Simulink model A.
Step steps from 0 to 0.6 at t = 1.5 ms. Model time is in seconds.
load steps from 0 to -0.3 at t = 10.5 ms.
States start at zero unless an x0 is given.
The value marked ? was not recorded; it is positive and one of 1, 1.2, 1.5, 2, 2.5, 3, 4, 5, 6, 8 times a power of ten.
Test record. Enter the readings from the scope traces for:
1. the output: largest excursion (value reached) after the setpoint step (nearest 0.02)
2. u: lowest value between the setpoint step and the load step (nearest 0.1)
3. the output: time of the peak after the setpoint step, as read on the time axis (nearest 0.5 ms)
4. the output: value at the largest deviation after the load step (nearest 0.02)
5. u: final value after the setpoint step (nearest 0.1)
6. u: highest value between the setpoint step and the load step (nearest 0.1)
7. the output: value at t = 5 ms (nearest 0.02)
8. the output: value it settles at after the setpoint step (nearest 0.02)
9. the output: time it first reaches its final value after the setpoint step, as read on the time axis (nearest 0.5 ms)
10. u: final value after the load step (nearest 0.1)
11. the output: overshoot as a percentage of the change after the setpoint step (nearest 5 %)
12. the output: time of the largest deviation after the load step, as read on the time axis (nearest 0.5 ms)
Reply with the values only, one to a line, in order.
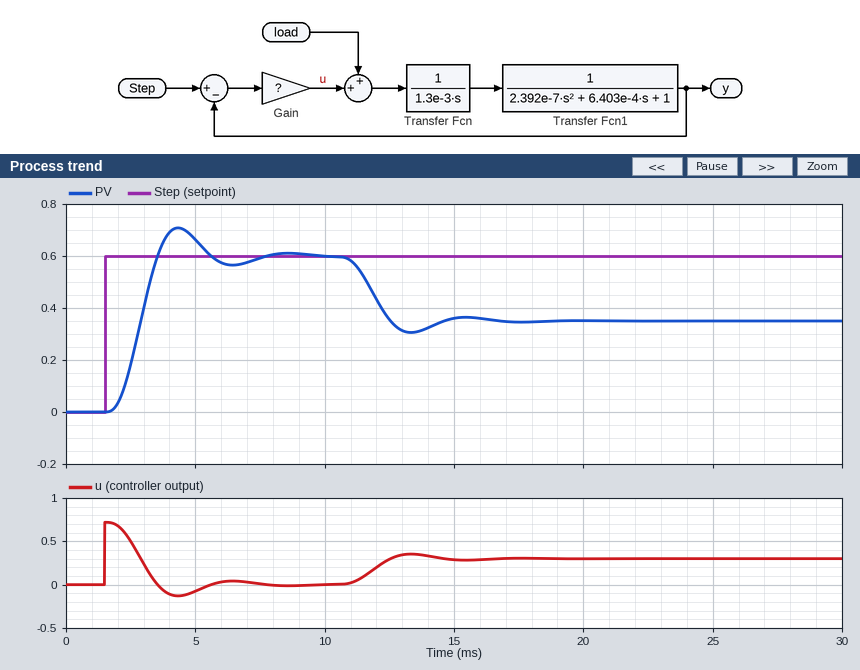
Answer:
0.70
-0.1
4.5 ms
0.30
0.0
0.7
0.66
0.60
3.5 ms
0.3
20 %
13.5 ms
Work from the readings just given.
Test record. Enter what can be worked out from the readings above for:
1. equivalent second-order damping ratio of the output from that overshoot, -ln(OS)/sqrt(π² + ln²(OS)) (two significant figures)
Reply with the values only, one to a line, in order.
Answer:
0.46
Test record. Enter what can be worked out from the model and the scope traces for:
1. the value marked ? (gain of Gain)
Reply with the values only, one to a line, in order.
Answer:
1.2
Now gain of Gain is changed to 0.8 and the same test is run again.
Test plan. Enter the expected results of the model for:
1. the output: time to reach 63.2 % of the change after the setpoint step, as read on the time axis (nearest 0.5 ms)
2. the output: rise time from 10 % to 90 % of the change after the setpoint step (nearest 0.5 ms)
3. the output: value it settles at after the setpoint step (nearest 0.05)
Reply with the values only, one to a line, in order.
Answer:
3.5 ms
2.0 ms
0.60
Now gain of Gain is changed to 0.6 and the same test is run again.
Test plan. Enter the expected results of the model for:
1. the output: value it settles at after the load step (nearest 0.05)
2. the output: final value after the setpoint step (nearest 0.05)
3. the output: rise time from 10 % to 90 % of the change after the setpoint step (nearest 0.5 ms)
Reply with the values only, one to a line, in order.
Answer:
0.10
0.60
3.0 ms
